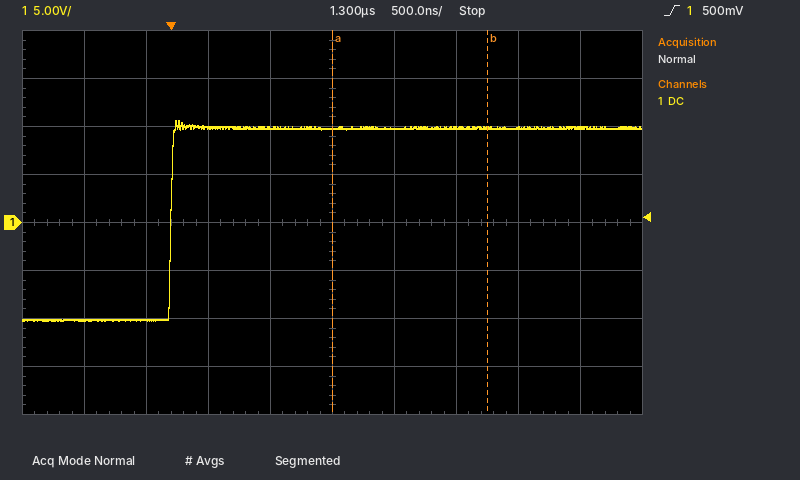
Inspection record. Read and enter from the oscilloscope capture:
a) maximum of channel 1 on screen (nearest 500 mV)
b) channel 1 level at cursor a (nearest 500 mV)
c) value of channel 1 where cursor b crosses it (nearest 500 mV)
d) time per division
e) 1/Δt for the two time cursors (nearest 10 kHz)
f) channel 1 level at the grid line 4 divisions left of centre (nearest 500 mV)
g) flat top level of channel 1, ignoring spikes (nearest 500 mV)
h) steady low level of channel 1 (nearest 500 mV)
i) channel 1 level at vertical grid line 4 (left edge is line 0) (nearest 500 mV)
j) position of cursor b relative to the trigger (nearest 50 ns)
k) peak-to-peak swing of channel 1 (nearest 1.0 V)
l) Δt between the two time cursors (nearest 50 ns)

10.5 V
10.0 V
10.0 V
500 ns
800 kHz
-10.0 V
10.0 V
-10.0 V
10.0 V
+2.55 µs
21.0 V
1.25 µs
